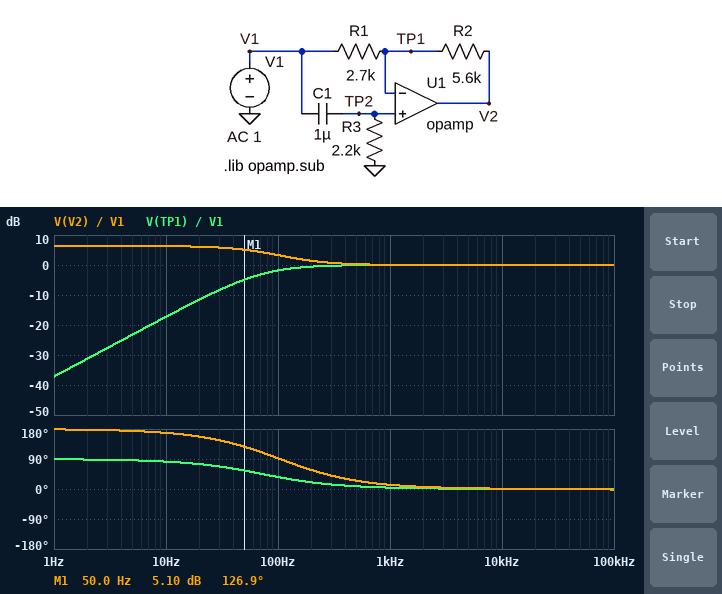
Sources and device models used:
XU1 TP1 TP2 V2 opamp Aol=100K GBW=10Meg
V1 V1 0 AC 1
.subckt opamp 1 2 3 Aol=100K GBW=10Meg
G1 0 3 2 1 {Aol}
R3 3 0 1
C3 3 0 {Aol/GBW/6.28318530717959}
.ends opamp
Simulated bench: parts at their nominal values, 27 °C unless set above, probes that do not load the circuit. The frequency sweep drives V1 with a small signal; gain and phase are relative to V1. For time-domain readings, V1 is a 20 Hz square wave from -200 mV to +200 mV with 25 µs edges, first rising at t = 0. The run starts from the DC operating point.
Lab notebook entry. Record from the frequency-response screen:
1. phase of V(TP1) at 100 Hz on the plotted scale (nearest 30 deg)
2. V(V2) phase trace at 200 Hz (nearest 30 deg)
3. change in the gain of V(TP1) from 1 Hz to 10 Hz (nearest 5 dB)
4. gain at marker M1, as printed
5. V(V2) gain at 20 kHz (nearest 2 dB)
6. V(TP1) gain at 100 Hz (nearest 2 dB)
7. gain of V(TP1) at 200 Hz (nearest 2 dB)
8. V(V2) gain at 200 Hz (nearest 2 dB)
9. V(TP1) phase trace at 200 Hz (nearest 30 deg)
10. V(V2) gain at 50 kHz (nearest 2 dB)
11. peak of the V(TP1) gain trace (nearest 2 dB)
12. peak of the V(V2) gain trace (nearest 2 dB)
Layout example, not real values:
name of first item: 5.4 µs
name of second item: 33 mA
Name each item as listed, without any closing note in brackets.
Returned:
phase of V(TP1) at 100 Hz on the plotted scale: 30 deg
V(V2) phase trace at 200 Hz: 60 deg
change in the gain of V(TP1) from 1 Hz to 10 Hz: 20 dB
gain at marker M1, as printed: 5.10 dB
V(V2) gain at 20 kHz: 0 dB
V(TP1) gain at 100 Hz: -2 dB
gain of V(TP1) at 200 Hz: 0 dB
V(V2) gain at 200 Hz: 2 dB
V(TP1) phase trace at 200 Hz: 30 deg
V(V2) gain at 50 kHz: 0 dB
peak of the V(TP1) gain trace: 0 dB
peak of the V(V2) gain trace: 6 dB
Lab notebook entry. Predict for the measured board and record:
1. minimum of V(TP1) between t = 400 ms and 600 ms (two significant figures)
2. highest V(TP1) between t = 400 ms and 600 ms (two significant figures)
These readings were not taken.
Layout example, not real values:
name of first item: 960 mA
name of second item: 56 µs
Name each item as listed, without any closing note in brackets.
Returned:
minimum of V(TP1) between t = 400 ms and 600 ms: -400 mV
highest V(TP1) between t = 400 ms and 600 ms: 400 mV
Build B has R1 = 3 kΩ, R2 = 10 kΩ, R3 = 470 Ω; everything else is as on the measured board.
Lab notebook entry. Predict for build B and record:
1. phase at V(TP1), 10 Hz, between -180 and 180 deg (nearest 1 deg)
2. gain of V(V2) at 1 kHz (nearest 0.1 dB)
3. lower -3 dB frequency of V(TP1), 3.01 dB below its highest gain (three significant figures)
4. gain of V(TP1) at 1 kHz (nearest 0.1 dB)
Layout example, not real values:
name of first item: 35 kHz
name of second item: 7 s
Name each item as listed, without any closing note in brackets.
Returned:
phase at V(TP1), 10 Hz, between -180 and 180 deg: 88 deg
gain of V(V2) at 1 kHz: 3.1 dB
lower -3 dB frequency of V(TP1), 3.01 dB below its highest gain: 339 Hz
gain of V(TP1) at 1 kHz: -0.5 dB
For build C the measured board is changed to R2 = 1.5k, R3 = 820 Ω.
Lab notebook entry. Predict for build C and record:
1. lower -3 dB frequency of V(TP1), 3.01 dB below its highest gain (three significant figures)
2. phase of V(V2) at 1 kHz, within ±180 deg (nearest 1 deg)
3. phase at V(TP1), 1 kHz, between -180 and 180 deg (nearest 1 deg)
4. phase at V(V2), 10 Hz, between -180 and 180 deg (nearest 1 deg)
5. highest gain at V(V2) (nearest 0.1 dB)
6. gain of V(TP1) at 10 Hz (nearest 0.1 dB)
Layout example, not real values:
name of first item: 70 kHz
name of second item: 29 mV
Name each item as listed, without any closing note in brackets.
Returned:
lower -3 dB frequency of V(TP1), 3.01 dB below its highest gain: 194 Hz
phase of V(V2) at 1 kHz, within ±180 deg: 17 deg
phase at V(TP1), 1 kHz, between -180 and 180 deg: 11 deg
phase at V(V2), 10 Hz, between -180 and 180 deg: 172 deg
highest gain at V(V2): 0 dB
gain of V(TP1) at 10 Hz: -25.8 dB
